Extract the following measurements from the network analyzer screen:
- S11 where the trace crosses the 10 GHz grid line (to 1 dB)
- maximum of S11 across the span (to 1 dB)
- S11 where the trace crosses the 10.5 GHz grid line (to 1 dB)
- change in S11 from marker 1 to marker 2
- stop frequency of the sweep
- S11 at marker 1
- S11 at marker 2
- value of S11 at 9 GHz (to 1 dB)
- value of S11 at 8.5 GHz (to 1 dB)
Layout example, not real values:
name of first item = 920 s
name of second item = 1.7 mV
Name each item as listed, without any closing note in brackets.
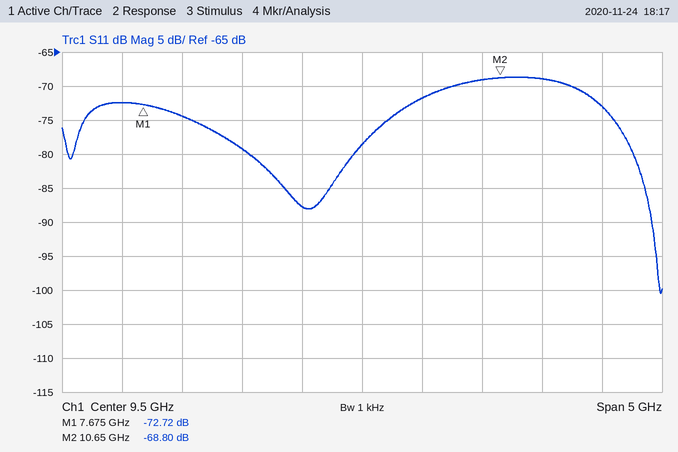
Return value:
S11 where the trace crosses the 10 GHz grid line = -72 dB
maximum of S11 across the span = -69 dB
S11 where the trace crosses the 10.5 GHz grid line = -69 dB
change in S11 from marker 1 to marker 2 = 3.92 dB
stop frequency of the sweep = 12 GHz
S11 at marker 1 = -72.72 dB
S11 at marker 2 = -68.80 dB
value of S11 at 9 GHz = -88 dB
value of S11 at 8.5 GHz = -79 dB
